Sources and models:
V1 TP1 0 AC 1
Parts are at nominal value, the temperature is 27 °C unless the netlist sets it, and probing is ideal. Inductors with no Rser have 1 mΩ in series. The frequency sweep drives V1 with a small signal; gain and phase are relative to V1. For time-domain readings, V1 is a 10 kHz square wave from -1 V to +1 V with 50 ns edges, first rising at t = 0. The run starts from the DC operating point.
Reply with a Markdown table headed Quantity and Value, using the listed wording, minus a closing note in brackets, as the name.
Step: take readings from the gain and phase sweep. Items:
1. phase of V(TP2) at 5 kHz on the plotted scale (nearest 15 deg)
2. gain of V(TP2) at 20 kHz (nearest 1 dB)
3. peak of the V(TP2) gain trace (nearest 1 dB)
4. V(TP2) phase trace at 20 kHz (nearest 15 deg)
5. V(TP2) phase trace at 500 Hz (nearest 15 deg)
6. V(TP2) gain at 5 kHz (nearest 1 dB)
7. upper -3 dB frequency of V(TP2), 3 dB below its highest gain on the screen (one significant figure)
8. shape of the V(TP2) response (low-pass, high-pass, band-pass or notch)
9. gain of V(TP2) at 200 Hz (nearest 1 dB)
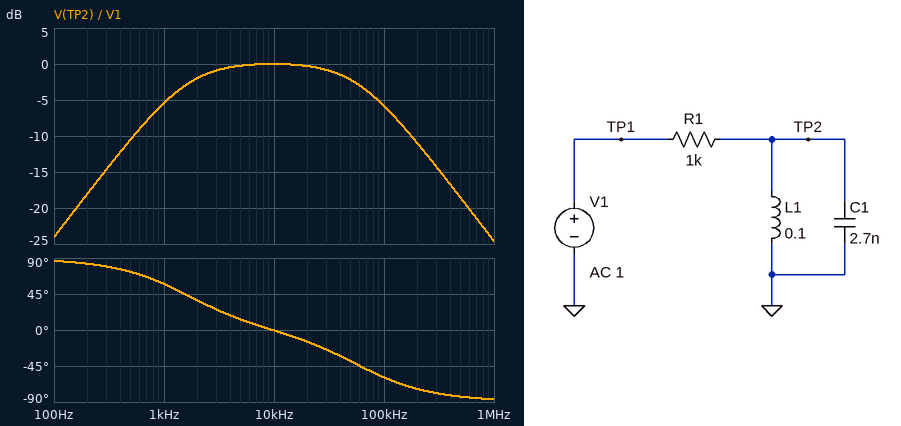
| Quantity | Value |
|---|---|
| phase of V(TP2) at 5 kHz on the plotted scale | 15 deg |
| gain of V(TP2) at 20 kHz | 0 dB |
| peak of the V(TP2) gain trace | 0 dB |
| V(TP2) phase trace at 20 kHz | -15 deg |
| V(TP2) phase trace at 500 Hz | 75 deg |
| V(TP2) gain at 5 kHz | 0 dB |
| upper -3 dB frequency of V(TP2), 3 dB below its highest gain on the screen | 60 kHz |
| shape of the V(TP2) response | band-pass |
| gain of V(TP2) at 200 Hz | -18 dB |
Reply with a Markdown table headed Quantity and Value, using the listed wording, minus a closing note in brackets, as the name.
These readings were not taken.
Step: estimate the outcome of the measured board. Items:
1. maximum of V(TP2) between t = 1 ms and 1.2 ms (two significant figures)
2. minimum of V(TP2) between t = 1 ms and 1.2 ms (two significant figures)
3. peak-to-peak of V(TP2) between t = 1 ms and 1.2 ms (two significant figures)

| Quantity | Value |
|---|---|
| maximum of V(TP2) between t = 1 ms and 1.2 ms | 1.1 V |
| minimum of V(TP2) between t = 1 ms and 1.2 ms | -1.1 V |
| peak-to-peak of V(TP2) between t = 1 ms and 1.2 ms | 2.3 V |
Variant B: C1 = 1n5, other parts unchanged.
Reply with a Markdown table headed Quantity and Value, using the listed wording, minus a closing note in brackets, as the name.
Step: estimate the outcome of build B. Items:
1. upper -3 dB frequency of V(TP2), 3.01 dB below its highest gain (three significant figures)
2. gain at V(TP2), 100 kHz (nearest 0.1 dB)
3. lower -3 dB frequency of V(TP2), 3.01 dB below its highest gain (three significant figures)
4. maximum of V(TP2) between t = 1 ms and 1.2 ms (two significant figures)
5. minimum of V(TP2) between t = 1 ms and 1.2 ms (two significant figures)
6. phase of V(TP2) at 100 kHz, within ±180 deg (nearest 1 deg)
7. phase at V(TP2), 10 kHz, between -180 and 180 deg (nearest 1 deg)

| Quantity | Value |
|---|---|
| upper -3 dB frequency of V(TP2), 3.01 dB below its highest gain | 108 kHz |
| gain at V(TP2), 100 kHz | -2.7 dB |
| lower -3 dB frequency of V(TP2), 3.01 dB below its highest gain | 1.57 kHz |
| maximum of V(TP2) between t = 1 ms and 1.2 ms | 1.2 V |
| minimum of V(TP2) between t = 1 ms and 1.2 ms | -1.2 V |
| phase of V(TP2) at 100 kHz, within ±180 deg | -43 deg |
| phase at V(TP2), 10 kHz, between -180 and 180 deg | 4 deg |
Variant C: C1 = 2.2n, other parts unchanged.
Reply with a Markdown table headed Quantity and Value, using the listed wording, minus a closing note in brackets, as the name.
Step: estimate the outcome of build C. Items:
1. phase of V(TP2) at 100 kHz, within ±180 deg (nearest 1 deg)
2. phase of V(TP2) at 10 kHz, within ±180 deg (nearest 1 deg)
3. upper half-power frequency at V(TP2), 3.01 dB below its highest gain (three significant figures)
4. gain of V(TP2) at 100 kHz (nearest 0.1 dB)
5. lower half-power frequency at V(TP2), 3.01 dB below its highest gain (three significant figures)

| Quantity | Value |
|---|---|
| phase of V(TP2) at 100 kHz, within ±180 deg | -54 deg |
| phase of V(TP2) at 10 kHz, within ±180 deg | 1 deg |
| upper half-power frequency at V(TP2), 3.01 dB below its highest gain | 73.9 kHz |
| gain of V(TP2) at 100 kHz | -4.6 dB |
| lower half-power frequency at V(TP2), 3.01 dB below its highest gain | 1.56 kHz |
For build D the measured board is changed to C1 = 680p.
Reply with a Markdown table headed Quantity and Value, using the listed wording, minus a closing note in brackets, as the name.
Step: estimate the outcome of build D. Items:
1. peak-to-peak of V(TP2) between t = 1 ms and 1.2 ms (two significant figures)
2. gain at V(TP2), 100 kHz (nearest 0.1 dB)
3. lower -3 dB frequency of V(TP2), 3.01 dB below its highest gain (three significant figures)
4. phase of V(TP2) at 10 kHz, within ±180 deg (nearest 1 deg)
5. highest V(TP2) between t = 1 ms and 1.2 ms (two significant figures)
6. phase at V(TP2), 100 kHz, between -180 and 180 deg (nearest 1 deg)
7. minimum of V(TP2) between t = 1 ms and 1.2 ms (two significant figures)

| Quantity | Value |
|---|---|
| peak-to-peak of V(TP2) between t = 1 ms and 1.2 ms | 2.4 V |
| gain at V(TP2), 100 kHz | -0.7 dB |
| lower -3 dB frequency of V(TP2), 3.01 dB below its highest gain | 1.58 kHz |
| phase of V(TP2) at 10 kHz, within ±180 deg | 7 deg |
| highest V(TP2) between t = 1 ms and 1.2 ms | 1.2 V |
| phase at V(TP2), 100 kHz, between -180 and 180 deg | -22 deg |
| minimum of V(TP2) between t = 1 ms and 1.2 ms | -1.2 V |
